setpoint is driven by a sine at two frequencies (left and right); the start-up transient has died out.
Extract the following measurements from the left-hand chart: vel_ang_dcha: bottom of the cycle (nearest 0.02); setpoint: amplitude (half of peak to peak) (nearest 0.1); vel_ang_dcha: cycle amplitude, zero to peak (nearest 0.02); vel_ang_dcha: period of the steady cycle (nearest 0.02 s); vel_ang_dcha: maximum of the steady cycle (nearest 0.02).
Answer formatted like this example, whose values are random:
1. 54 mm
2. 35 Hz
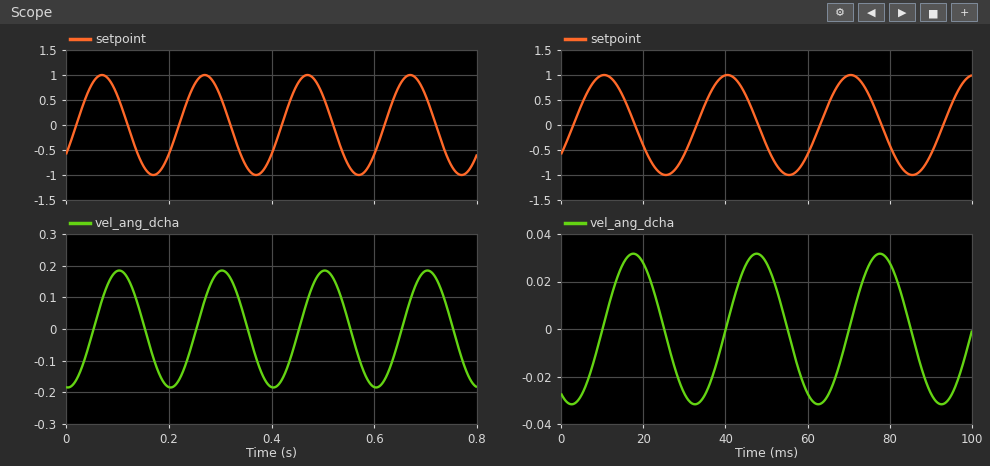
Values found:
1. -0.18
2. 1.0
3. 0.18
4. 0.20 s
5. 0.18
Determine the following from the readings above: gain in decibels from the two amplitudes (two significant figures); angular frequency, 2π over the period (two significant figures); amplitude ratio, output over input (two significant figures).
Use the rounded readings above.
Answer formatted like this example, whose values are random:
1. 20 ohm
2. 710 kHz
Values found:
1. -15 dB
2. 31 rad/s
3. 0.18
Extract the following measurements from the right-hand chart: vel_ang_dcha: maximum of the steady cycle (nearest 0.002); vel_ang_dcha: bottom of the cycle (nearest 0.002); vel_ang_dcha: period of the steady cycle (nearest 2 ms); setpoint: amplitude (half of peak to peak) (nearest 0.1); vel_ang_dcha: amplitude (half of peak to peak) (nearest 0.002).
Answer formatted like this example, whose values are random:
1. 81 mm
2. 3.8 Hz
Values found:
1. 0.032
2. -0.032
3. 30 ms
4. 1.0
5. 0.032
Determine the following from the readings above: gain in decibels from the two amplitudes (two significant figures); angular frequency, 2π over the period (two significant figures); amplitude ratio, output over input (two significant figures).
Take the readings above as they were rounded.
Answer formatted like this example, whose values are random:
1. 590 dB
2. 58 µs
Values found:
1. -30 dB
2. 0.21 rad/ms
3. 0.032
